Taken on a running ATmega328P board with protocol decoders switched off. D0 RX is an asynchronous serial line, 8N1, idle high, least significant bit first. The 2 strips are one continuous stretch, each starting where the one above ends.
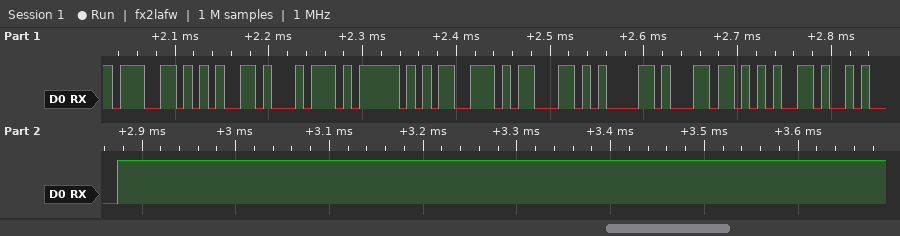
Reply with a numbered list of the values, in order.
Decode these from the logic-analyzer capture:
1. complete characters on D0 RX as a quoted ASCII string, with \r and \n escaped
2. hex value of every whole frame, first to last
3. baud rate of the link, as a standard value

1. "get_scale\n"
2. 67 65 74 5F 73 63 61 6C 65 0A
3. 115200 baud
